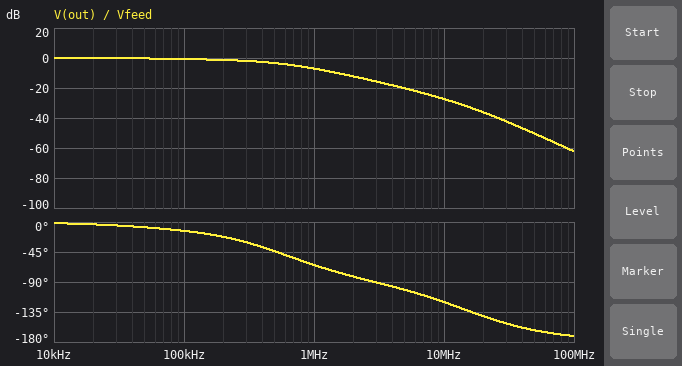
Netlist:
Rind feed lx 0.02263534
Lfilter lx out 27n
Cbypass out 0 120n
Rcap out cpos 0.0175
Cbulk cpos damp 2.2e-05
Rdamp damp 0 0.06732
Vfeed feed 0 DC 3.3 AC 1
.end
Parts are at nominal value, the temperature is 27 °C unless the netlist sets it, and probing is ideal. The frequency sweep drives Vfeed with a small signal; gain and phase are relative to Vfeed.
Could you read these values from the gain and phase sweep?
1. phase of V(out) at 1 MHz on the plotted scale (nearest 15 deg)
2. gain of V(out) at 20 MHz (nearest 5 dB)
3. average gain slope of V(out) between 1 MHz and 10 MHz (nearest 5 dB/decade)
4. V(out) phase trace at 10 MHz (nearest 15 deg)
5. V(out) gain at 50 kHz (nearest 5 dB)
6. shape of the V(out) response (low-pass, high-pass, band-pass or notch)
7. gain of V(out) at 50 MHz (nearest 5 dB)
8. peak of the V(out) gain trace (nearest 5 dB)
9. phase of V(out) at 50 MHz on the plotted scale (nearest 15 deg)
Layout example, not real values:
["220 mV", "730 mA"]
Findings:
["-60 deg", "-35 dB", "-20 dB/decade", "-120 deg", "0 dB", "low-pass", "-50 dB", "0 dB", "-165 deg"]
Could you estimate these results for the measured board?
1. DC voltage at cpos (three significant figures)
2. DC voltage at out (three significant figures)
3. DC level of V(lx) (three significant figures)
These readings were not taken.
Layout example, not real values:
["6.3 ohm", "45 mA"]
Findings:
["3.30 V", "3.30 V", "3.30 V"]
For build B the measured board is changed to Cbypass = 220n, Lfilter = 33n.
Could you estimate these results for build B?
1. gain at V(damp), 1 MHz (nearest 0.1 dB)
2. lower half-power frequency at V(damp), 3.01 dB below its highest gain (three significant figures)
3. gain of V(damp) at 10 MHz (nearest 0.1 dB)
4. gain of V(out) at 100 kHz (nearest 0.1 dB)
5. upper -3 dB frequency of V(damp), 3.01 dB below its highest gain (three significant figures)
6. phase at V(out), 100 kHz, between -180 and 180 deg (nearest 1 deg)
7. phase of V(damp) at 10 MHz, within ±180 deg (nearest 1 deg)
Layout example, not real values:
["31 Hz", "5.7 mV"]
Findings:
["-10.3 dB", "60.8 kHz", "-33.4 dB", "-0.6 dB", "595 kHz", "-15 deg", "-138 deg"]
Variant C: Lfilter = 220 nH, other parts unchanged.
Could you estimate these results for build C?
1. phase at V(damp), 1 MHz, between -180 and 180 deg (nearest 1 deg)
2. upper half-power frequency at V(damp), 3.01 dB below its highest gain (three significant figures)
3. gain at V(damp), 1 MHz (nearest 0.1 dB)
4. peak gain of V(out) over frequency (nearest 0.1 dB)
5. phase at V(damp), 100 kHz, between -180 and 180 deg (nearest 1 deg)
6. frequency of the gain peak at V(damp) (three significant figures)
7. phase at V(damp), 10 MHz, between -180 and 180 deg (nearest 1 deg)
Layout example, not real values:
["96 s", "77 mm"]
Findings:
["-89 deg", "121 kHz", "-26.3 dB", "2.3 dB", "-32 deg", "72.3 kHz", "-122 deg"]
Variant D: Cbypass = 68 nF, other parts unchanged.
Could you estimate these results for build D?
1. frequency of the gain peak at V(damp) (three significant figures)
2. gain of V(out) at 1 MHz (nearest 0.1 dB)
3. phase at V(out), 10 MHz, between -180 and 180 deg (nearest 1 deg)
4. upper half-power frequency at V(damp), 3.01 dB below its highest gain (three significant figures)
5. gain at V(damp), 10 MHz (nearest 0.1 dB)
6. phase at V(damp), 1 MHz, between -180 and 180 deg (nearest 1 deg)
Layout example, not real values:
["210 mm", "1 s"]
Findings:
["208 kHz", "-7.1 dB", "-107 deg", "703 kHz", "-28.5 dB", "-58 deg"]
